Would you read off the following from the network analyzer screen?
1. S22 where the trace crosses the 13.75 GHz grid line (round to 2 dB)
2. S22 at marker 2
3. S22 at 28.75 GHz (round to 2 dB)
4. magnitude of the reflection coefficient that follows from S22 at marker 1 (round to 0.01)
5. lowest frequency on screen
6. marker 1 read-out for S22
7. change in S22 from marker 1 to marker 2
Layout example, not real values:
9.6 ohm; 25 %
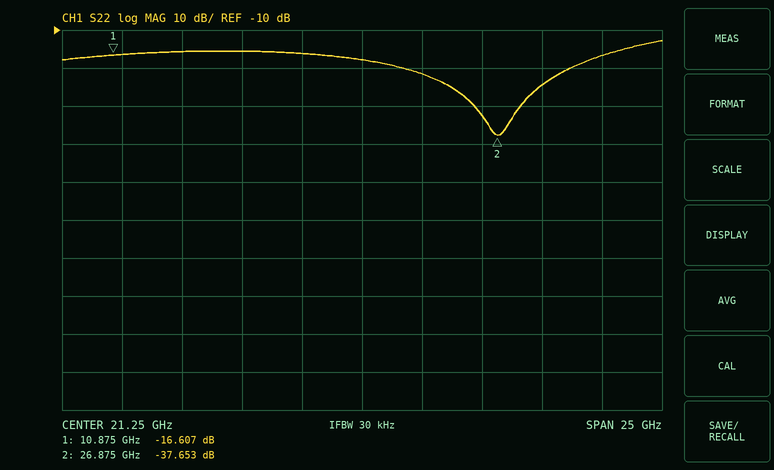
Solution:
-16 dB; -37.653 dB; -24 dB; 0.15; 8.75 GHz; -16.607 dB; -21.046 dB
